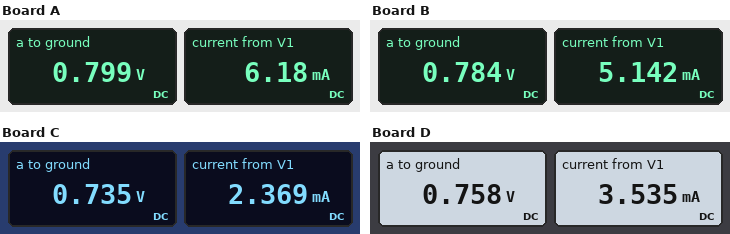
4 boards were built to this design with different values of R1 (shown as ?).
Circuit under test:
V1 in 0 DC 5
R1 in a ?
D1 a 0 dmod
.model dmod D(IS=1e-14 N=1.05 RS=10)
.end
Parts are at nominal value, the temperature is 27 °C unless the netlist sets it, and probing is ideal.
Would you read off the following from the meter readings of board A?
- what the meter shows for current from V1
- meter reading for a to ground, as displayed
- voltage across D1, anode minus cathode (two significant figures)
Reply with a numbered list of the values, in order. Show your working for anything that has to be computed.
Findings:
1. 6.18 mA
2. 0.799 V
3. 799 mV = 800 mV
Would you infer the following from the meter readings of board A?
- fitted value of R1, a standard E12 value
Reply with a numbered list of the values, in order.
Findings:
1. 680 Ω
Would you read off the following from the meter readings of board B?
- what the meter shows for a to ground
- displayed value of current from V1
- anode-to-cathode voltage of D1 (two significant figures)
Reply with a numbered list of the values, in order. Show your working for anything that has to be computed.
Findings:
1. 0.784 V
2. 5.142 mA
3. 784 mV = 780 mV
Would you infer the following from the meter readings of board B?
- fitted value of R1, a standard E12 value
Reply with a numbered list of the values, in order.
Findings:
1. 820 Ω
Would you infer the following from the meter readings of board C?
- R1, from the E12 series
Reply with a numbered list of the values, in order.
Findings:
1. 1.8 kΩ
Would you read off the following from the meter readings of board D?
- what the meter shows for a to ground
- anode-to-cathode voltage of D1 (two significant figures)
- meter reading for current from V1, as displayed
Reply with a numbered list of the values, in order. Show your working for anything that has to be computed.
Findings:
1. 0.758 V
2. 758 mV = 760 mV
3. 3.535 mA
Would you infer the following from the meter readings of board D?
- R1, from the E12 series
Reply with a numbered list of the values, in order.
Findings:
1. 1.2 kΩ
